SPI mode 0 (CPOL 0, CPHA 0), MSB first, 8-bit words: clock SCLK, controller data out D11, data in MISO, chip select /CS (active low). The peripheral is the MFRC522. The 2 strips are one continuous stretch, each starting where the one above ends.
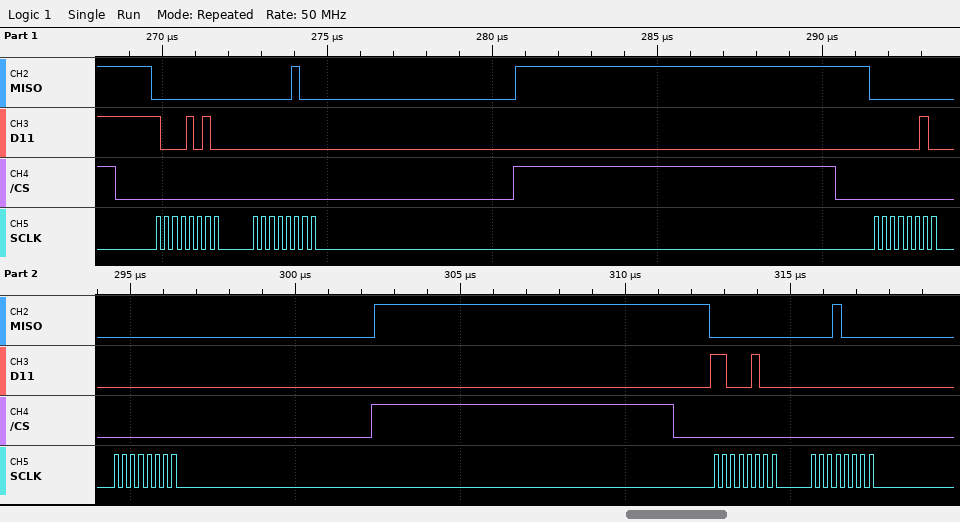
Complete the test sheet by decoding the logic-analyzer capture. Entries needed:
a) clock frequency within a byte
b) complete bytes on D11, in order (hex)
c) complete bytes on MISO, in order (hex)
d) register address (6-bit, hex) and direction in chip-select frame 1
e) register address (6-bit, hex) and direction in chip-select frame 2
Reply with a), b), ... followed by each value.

a) 4 MHz
b) 8A 00 02 00 C4 00
c) 00 04 00 00 00 10
d) 0x05 read
e) 0x01 write
